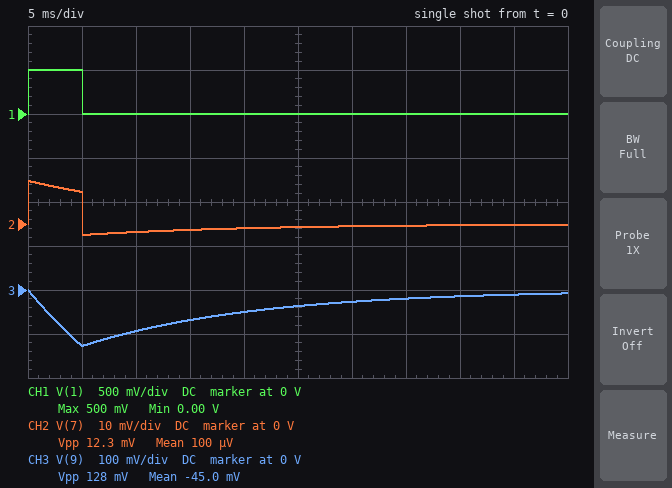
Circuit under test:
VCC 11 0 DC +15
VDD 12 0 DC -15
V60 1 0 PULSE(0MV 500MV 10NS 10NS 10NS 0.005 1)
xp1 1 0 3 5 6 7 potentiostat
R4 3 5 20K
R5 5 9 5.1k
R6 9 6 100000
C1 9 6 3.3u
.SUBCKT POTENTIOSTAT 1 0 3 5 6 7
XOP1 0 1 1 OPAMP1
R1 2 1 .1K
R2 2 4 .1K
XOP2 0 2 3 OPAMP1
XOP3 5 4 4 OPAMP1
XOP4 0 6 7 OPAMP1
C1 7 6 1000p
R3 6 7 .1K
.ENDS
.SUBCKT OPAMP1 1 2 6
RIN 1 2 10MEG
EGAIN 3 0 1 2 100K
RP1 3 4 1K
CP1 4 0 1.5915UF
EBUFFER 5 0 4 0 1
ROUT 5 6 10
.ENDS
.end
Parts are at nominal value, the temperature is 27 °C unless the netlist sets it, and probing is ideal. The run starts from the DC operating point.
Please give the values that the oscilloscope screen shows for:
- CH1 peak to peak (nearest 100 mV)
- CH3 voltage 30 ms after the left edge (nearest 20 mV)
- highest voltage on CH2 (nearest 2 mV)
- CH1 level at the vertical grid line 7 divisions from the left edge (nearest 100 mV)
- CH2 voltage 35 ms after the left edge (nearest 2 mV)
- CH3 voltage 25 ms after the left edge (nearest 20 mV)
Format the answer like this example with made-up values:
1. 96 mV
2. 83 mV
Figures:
1. 500 mV
2. -20 mV
3. 10 mV
4. 0 V
5. 0 V
6. -40 mV
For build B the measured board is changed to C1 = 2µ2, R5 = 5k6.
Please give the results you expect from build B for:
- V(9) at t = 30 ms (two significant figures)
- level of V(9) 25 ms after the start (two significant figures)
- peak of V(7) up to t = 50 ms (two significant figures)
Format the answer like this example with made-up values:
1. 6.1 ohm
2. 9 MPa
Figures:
1. -19 mV
2. -30 mV
3. 8.9 mV
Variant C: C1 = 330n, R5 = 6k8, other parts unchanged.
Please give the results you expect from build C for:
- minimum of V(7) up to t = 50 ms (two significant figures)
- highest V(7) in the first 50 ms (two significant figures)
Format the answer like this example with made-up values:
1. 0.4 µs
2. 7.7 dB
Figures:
1. -6.2 mV
2. 7.4 mV
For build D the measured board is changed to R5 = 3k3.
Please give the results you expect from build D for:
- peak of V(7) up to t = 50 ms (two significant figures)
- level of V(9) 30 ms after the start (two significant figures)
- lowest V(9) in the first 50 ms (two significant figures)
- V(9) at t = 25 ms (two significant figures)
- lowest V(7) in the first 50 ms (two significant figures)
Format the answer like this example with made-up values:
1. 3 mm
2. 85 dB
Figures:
1. 15 mV
2. -17 mV
3. -180 mV
4. -27 mV
5. -5.5 mV
